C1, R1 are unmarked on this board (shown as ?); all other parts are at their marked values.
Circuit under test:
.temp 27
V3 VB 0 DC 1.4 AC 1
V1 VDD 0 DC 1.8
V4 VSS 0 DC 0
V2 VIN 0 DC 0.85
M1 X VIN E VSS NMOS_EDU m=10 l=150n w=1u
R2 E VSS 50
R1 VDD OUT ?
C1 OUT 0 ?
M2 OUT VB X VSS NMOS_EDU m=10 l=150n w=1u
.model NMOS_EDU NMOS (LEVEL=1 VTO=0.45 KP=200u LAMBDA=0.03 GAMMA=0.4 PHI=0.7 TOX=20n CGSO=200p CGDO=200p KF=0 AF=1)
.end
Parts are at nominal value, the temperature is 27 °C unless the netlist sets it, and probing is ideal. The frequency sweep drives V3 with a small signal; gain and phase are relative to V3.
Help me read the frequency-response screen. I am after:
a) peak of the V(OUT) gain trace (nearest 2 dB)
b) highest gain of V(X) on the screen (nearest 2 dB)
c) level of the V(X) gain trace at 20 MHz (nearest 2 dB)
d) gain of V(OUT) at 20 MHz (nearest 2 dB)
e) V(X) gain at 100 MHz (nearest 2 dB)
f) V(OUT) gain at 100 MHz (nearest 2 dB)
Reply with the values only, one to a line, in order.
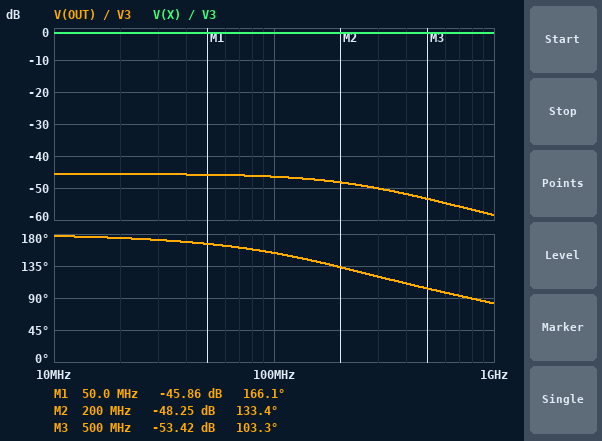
-46 dB
-2 dB
-2 dB
-46 dB
-2 dB
-46 dB
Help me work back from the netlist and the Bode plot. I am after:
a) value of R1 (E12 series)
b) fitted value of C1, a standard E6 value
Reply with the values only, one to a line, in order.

330 Ω
2.2 pF
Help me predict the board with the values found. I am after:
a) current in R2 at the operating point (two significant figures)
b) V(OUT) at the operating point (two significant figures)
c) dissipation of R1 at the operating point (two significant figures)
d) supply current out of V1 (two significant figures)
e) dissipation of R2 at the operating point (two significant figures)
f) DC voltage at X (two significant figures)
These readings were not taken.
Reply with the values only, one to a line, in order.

820 µA
1.5 V
220 µW
820 µA
34 µW
500 mV
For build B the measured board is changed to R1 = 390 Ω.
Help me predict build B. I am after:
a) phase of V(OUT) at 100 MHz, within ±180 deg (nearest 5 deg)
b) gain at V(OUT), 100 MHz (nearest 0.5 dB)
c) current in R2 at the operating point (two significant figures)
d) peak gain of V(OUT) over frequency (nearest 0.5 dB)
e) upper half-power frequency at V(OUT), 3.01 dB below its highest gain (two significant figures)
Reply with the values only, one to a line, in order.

150 deg
-45.5 dB
820 µA
-44.0 dB
190 MHz
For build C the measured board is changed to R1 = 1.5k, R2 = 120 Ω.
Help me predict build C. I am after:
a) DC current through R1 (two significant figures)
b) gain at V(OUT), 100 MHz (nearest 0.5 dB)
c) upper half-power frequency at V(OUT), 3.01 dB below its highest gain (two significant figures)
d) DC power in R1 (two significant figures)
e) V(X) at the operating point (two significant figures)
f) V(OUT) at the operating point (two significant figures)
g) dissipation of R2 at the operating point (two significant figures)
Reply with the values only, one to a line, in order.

630 µA
-44.0 dB
48 MHz
600 µW
530 mV
850 mV
48 µW
